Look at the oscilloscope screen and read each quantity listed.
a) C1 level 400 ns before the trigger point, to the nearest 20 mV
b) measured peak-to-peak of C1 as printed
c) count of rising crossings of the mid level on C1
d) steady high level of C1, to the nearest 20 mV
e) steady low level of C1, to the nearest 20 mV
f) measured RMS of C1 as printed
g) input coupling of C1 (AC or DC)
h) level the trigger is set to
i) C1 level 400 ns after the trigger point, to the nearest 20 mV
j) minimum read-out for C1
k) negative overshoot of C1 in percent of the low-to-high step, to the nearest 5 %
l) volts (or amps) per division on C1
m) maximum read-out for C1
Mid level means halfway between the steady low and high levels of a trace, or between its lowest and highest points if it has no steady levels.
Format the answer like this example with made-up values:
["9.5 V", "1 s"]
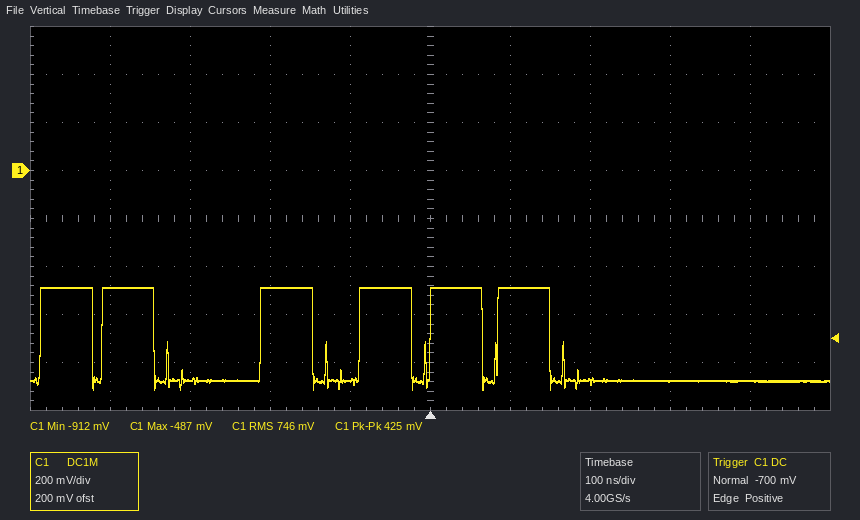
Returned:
["-480 mV", "425 mV", "6", "-480 mV", "-880 mV", "746 mV", "DC", "-700 mV", "-880 mV", "-912 mV", "10 %", "200 mV", "-487 mV"]
